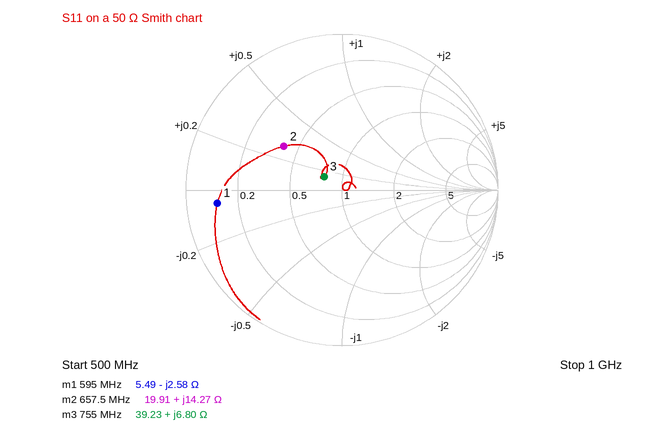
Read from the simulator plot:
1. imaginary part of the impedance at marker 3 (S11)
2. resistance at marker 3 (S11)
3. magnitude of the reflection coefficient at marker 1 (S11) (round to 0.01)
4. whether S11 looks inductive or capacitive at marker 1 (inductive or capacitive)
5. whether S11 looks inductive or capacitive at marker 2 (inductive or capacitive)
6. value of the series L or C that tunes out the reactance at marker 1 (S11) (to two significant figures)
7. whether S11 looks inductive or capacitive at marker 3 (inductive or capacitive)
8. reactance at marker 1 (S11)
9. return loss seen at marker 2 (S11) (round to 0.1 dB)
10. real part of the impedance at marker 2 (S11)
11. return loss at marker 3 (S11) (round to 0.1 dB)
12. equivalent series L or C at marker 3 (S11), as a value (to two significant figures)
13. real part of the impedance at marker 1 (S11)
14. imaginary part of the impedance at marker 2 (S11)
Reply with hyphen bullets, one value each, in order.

- +6.80 Ω
- 39.23 Ω
- 0.80
- capacitive
- inductive
- 690 pH
- inductive
- -2.58 Ω
- 6.6 dB
- 19.91 Ω
- 16.9 dB
- 1.4 nH
- 5.49 Ω
- +14.27 Ω
